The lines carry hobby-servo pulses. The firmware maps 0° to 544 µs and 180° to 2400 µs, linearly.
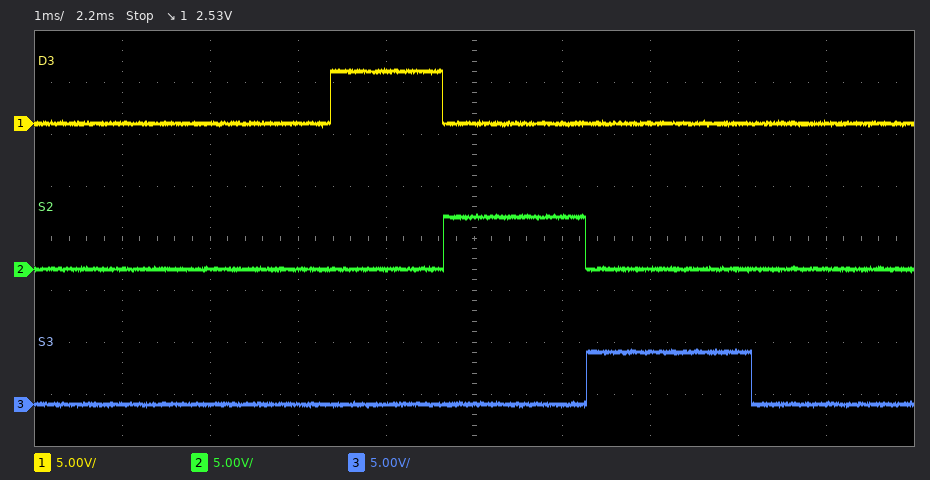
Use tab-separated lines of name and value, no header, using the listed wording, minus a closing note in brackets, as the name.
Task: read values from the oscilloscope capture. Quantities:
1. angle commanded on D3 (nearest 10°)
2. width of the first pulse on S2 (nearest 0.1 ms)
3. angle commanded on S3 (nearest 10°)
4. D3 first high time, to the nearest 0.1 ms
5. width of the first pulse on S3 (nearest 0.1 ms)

angle commanded on D3	70°
width of the first pulse on S2	1.6 ms
angle commanded on S3	130°
D3 first high time, to the nearest 0.1 ms	1.3 ms
width of the first pulse on S3	1.9 ms
